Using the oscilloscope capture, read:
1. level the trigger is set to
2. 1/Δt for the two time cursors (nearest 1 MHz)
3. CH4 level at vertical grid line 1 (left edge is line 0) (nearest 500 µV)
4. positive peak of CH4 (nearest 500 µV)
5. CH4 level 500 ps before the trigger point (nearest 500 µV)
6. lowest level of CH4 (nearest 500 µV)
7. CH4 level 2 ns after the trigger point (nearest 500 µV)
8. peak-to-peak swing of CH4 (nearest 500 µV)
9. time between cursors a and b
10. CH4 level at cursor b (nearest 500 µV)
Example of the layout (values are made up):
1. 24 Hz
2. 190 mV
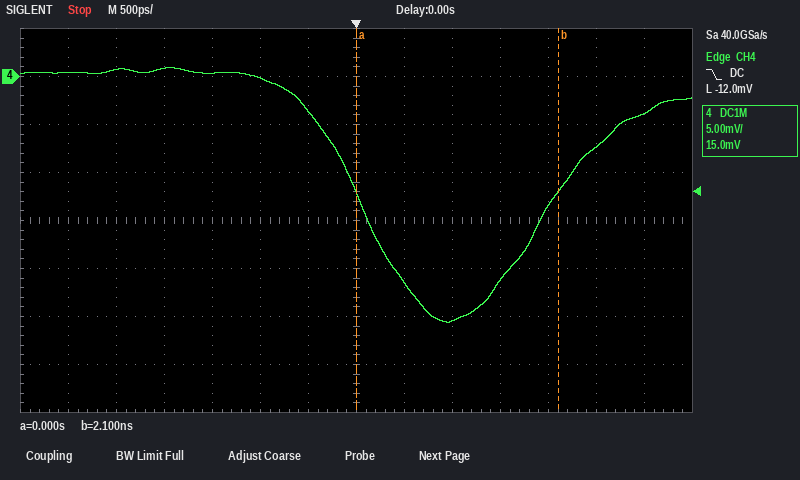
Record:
1. -12.0 mV
2. 476 MHz
3. 500 µV
4. 1.0 mV
5. -3.5 mV
6. -25.5 mV
7. -13.5 mV
8. 26.5 mV
9. 2.10 ns
10. -12.0 mV
